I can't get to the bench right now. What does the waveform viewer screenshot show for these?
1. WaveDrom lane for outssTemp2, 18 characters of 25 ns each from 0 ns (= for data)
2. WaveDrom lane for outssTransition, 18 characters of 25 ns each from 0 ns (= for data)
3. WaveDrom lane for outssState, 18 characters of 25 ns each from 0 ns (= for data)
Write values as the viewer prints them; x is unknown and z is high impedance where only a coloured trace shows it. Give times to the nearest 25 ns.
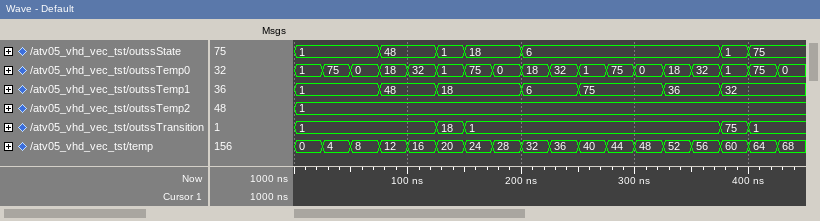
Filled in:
{name: 'outssTemp2', wave: '=.................', data: '1'}
{name: 'outssTransition', wave: '=....==........==.', data: '1 18 1 75 1'}
{name: 'outssState', wave: '=..=.==.=......==.', data: '1 48 1 18 6 1 75'}
